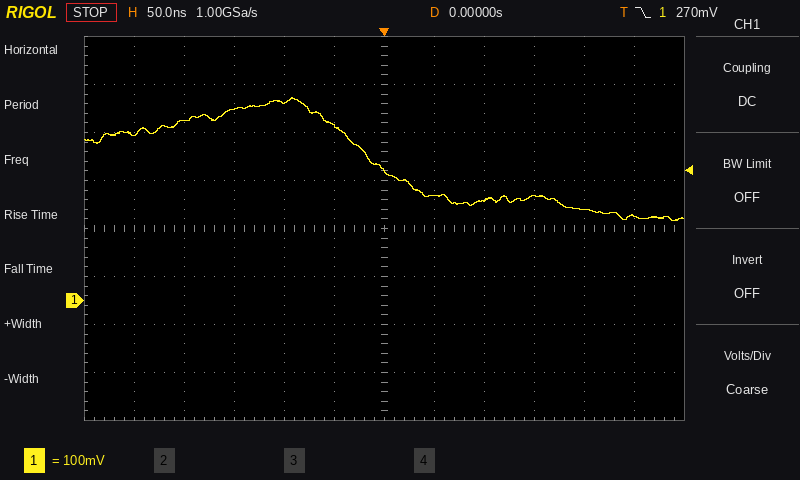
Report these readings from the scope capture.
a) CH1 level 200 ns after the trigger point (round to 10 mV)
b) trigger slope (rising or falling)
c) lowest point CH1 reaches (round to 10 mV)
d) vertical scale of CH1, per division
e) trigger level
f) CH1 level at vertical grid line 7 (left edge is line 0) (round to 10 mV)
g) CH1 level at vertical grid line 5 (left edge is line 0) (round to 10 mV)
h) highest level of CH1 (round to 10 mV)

190 mV
falling
170 mV
100 mV
270 mV
220 mV
360 mV
420 mV
